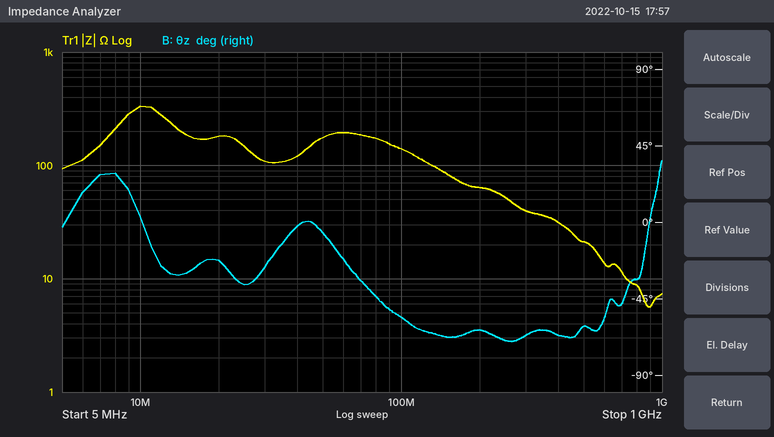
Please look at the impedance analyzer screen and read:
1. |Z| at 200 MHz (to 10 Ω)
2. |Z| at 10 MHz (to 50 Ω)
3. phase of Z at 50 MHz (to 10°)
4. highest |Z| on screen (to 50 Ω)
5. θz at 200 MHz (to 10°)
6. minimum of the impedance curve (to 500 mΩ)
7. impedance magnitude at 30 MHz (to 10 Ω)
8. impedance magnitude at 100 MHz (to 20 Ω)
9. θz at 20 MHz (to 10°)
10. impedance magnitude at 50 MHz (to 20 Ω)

60 Ω
350 Ω
-10°
350 Ω
-60°
5.5 Ω
110 Ω
140 Ω
-20°
180 Ω
